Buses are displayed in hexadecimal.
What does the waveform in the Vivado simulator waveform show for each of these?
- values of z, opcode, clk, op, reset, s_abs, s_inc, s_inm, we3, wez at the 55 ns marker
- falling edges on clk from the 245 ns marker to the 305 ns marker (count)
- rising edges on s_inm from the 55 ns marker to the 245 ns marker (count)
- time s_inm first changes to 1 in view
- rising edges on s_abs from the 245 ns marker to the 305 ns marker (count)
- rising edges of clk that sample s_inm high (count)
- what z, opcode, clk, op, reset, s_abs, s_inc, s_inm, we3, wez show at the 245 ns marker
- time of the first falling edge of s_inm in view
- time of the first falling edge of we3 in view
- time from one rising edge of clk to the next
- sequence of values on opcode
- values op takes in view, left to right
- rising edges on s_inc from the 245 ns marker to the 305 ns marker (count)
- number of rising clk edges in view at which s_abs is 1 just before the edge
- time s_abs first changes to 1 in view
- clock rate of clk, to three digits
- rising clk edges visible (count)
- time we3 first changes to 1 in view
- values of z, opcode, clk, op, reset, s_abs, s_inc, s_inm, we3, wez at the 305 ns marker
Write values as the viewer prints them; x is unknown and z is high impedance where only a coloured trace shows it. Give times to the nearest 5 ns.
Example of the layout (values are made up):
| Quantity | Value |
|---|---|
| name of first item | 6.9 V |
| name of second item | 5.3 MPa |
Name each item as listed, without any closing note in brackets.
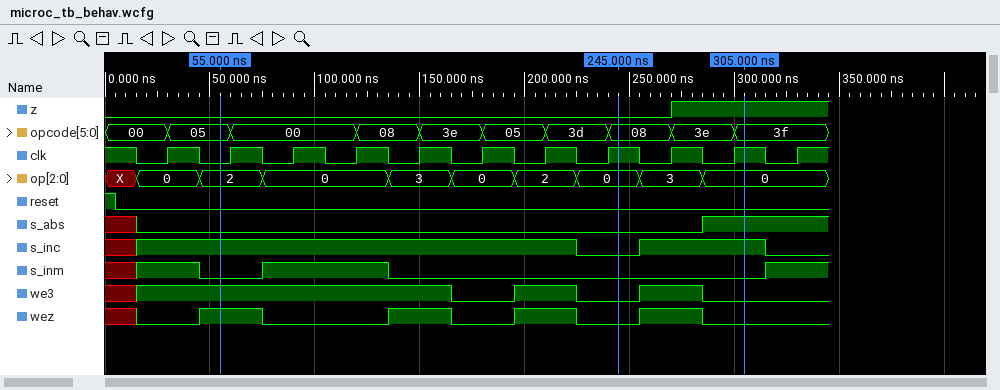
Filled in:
| Quantity | Value |
|---|---|
| values of z, opcode, clk, op, reset, s_abs, s_inc, s_inm, we3, wez at the 55 ns marker | z=0, opcode=05, clk=0, op=2, reset=0, s_abs=0, s_inc=1, s_inm=0, we3=1, wez=1 |
| falling edges on clk from the 245 ns marker to the 305 ns marker | 2 |
| rising edges on s_inm from the 55 ns marker to the 245 ns marker | 1 |
| time s_inm first changes to 1 in view | 15 ns |
| rising edges on s_abs from the 245 ns marker to the 305 ns marker | 1 |
| rising edges of clk that sample s_inm high | 4 |
| what z, opcode, clk, op, reset, s_abs, s_inc, s_inm, we3, wez show at the 245 ns marker | z=0, opcode=08, clk=1, op=0, reset=0, s_abs=0, s_inc=0, s_inm=0, we3=0, wez=0 |
| time of the first falling edge of s_inm in view | 45 ns |
| time of the first falling edge of we3 in view | 165 ns |
| time from one rising edge of clk to the next | 30 ns |
| sequence of values on opcode | 00, 05, 00, 08, 3e, 05, 3d, 08, 3e, 3f |
| values op takes in view, left to right | X, 0, 2, 0, 3, 0, 2, 0, 3, 0 |
| rising edges on s_inc from the 245 ns marker to the 305 ns marker | 1 |
| number of rising clk edges in view at which s_abs is 1 just before the edge | 2 |
| time s_abs first changes to 1 in view | 285 ns |
| clock rate of clk, to three digits | 33.3 MHz |
| rising clk edges visible | 11 |
| time we3 first changes to 1 in view | 15 ns |
| values of z, opcode, clk, op, reset, s_abs, s_inc, s_inm, we3, wez at the 305 ns marker | z=1, opcode=3f, clk=1, op=0, reset=0, s_abs=1, s_inc=1, s_inm=0, we3=0, wez=0 |
